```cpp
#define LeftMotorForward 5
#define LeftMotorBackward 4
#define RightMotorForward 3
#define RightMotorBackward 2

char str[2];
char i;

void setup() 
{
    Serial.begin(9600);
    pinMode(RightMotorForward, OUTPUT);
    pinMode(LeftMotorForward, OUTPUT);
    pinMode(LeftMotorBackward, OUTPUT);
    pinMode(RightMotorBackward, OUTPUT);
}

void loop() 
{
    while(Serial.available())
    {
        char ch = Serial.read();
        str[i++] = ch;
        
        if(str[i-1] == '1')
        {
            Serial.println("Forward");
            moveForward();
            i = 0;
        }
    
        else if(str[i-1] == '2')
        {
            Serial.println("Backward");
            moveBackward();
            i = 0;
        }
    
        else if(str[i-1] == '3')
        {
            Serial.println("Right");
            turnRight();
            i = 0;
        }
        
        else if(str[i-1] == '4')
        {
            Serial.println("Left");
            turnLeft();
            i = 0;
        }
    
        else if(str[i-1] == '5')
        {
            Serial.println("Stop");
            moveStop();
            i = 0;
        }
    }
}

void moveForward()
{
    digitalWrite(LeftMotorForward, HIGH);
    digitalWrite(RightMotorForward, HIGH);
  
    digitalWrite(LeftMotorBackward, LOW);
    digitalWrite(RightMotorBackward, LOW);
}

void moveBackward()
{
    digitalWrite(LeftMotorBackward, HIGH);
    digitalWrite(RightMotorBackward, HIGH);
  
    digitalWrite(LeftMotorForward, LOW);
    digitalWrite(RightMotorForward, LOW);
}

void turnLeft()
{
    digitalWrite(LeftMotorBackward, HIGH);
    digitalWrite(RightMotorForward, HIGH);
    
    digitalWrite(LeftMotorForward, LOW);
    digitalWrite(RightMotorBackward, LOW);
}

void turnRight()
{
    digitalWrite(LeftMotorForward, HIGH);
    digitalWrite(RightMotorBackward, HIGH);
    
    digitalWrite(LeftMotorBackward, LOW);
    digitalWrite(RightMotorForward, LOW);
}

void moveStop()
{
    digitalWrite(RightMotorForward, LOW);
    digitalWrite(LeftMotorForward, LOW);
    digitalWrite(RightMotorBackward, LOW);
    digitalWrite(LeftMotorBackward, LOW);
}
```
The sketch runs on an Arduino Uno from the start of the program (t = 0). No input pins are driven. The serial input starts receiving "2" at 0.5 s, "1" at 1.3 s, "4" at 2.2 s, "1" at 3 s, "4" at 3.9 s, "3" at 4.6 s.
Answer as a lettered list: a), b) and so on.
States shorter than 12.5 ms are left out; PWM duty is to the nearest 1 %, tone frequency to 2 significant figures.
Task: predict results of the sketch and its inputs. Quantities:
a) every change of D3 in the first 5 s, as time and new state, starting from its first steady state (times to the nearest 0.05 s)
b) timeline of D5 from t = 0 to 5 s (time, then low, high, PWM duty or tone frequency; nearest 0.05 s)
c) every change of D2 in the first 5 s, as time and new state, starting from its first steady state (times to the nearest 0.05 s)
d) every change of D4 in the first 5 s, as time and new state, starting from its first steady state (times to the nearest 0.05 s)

a) 0 s low; 1.3 s high; 4.6 s low
b) 0 s low; 1.3 s high; 2.2 s low; 3 s high; 3.9 s low; 4.6 s high
c) 0 s low; 0.5 s high; 1.3 s low; 4.6 s high
d) 0 s low; 0.5 s high; 1.3 s low; 2.2 s high; 3 s low; 3.9 s high; 4.6 s low
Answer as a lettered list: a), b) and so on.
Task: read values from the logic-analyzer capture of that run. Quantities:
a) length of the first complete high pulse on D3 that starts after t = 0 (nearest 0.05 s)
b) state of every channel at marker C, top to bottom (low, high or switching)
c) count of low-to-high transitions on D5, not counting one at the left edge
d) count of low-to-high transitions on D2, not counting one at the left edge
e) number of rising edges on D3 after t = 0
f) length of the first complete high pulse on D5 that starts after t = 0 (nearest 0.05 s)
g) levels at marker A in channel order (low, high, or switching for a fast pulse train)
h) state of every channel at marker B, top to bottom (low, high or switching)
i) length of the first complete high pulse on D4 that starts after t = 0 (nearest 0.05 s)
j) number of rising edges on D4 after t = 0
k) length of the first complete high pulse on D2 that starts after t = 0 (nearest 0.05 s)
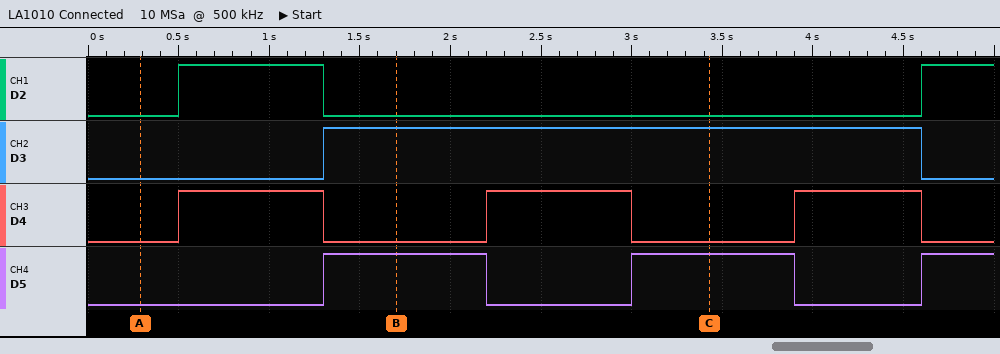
a) 3.30 s
b) D2 low, D3 high, D4 low, D5 high
c) 3
d) 2
e) 1
f) 0.90 s
g) D2 low, D3 low, D4 low, D5 low
h) D2 low, D3 high, D4 low, D5 high
i) 0.80 s
j) 3
k) 0.80 s
